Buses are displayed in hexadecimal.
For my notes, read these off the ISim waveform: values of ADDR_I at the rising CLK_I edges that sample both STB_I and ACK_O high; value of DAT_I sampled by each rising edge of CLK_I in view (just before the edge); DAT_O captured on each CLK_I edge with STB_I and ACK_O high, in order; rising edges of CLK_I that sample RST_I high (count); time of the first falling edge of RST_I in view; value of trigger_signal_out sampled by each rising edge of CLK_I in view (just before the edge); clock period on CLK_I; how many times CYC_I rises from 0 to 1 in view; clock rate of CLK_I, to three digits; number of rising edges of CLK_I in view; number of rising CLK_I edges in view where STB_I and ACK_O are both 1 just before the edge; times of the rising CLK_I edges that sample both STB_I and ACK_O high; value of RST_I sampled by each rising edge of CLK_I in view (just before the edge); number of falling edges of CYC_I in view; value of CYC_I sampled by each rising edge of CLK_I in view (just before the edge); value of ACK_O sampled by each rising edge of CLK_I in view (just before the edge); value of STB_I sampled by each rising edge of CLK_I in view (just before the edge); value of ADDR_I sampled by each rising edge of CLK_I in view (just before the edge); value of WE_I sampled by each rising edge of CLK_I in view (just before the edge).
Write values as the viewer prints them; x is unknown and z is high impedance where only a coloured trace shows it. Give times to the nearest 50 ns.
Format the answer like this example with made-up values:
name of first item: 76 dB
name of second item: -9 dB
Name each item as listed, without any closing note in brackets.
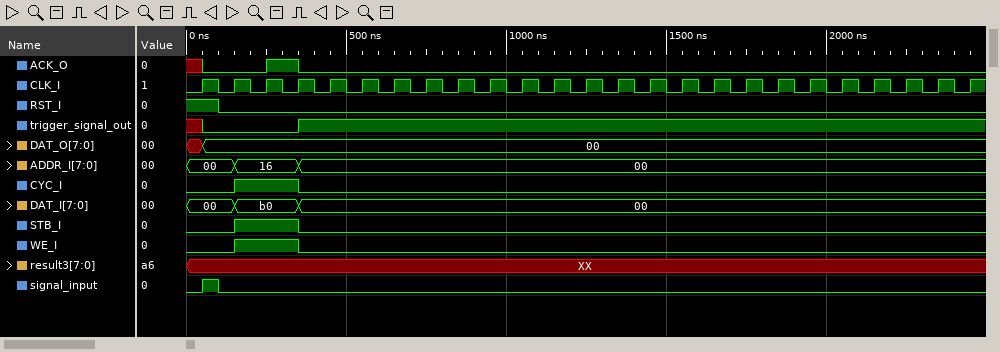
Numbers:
values of ADDR_I at the rising CLK_I edges that sample both STB_I and ACK_O high: 16
value of DAT_I sampled by each rising edge of CLK_I in view: 00, 00, b0, b0, 00, 00, 00, 00, 00, 00, 00, 00, 00, 00, 00, 00, 00, 00, 00, 00, 00, 00, 00, 00, 00
DAT_O captured on each CLK_I edge with STB_I and ACK_O high, in order: 00
rising edges of CLK_I that sample RST_I high: 1
time of the first falling edge of RST_I in view: 100 ns
value of trigger_signal_out sampled by each rising edge of CLK_I in view: x 0 0 0 1 1 1 1 1 1 1 1 1 1 1 1 1 1 1 1 1 1 1 1 1
clock period on CLK_I: 100 ns
how many times CYC_I rises from 0 to 1 in view: 1
clock rate of CLK_I, to three digits: 10.0 MHz
number of rising edges of CLK_I in view: 25
number of rising CLK_I edges in view where STB_I and ACK_O are both 1 just before the edge: 1
times of the rising CLK_I edges that sample both STB_I and ACK_O high: 350 ns
value of RST_I sampled by each rising edge of CLK_I in view: 1 0 0 0 0 0 0 0 0 0 0 0 0 0 0 0 0 0 0 0 0 0 0 0 0
number of falling edges of CYC_I in view: 1
value of CYC_I sampled by each rising edge of CLK_I in view: 0 0 1 1 0 0 0 0 0 0 0 0 0 0 0 0 0 0 0 0 0 0 0 0 0
value of ACK_O sampled by each rising edge of CLK_I in view: x 0 0 1 0 0 0 0 0 0 0 0 0 0 0 0 0 0 0 0 0 0 0 0 0
value of STB_I sampled by each rising edge of CLK_I in view: 0 0 1 1 0 0 0 0 0 0 0 0 0 0 0 0 0 0 0 0 0 0 0 0 0
value of ADDR_I sampled by each rising edge of CLK_I in view: 00, 00, 16, 16, 00, 00, 00, 00, 00, 00, 00, 00, 00, 00, 00, 00, 00, 00, 00, 00, 00, 00, 00, 00, 00
value of WE_I sampled by each rising edge of CLK_I in view: 0 0 1 1 0 0 0 0 0 0 0 0 0 0 0 0 0 0 0 0 0 0 0 0 0
